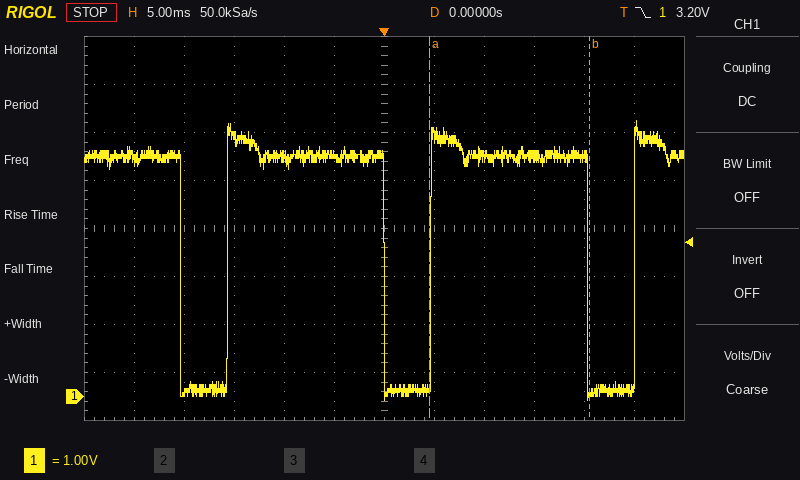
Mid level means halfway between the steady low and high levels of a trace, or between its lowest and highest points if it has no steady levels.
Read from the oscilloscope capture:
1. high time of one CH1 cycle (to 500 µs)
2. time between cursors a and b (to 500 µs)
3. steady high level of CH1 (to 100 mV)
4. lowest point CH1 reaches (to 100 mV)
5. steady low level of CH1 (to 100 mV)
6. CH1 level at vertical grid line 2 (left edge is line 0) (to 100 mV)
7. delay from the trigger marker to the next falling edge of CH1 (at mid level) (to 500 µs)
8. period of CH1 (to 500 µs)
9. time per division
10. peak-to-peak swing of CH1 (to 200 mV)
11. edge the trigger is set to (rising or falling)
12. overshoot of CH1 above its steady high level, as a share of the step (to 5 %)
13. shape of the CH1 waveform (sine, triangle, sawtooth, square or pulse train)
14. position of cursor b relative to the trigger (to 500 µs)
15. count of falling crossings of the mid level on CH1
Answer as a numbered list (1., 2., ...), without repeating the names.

1. 15.5 ms
2. 16.0 ms
3. 5.0 V
4. -100 mV
5. 100 mV
6. 100 mV
7. 20.5 ms
8. 20.5 ms
9. 5 ms
10. 5.8 V
11. falling
12. 15 %
13. pulse train
14. +20.5 ms
15. 3
